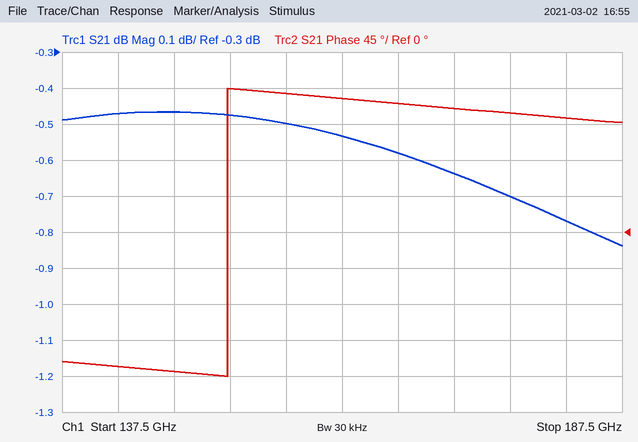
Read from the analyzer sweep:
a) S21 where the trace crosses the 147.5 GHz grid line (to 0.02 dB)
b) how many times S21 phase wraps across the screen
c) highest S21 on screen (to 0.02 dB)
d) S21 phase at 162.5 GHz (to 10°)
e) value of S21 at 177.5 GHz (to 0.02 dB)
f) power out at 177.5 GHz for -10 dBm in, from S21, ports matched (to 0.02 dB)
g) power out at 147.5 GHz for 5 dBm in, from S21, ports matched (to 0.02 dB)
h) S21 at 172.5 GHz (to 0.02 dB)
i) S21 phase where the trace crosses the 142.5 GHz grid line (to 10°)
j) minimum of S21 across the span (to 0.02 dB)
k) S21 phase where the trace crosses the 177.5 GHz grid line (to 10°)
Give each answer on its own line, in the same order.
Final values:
-0.46 dB
1
-0.46 dB
170°
-0.70 dB
-10.70 dBm
4.54 dBm
-0.64 dB
-170°
-0.84 dB
150°
